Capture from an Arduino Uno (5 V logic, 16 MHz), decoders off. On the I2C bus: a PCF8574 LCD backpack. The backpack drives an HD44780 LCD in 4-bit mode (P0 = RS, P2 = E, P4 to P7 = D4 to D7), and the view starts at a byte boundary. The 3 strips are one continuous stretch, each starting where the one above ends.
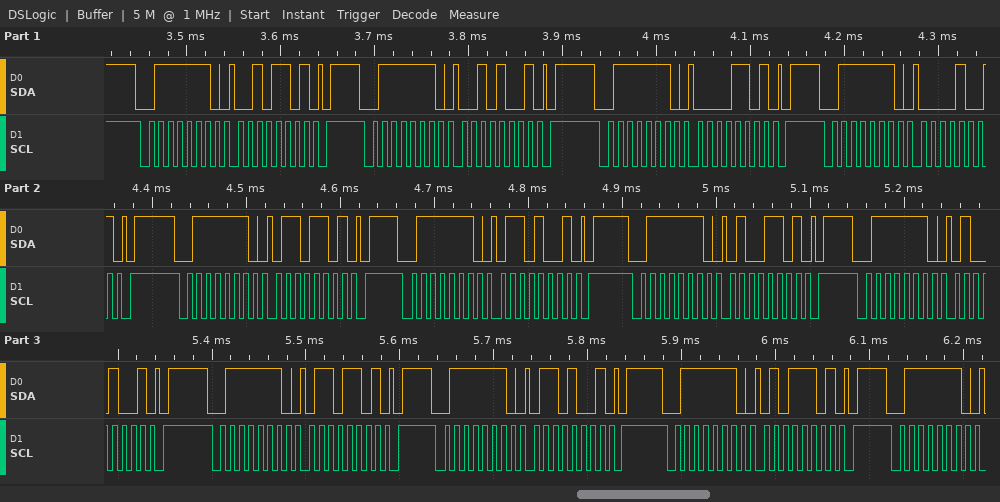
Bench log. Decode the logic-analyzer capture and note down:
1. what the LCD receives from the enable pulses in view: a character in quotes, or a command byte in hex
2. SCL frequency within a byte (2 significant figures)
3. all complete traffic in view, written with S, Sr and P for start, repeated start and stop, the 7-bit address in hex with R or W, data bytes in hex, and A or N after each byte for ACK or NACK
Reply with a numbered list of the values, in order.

1. ' ' 'd'
2. 100 kHz
3. S 3FW A 2D A P S 3FW A 29 A P S 3FW A 0D A P S 3FW A 09 A P S 3FW A 6D A P S 3FW A 69 A P S 3FW A 4D A P S 3FW A 49 A P S 3FW A 6D A P S 3FW A 69 A P S 3FW A 5D A P S 3FW A
